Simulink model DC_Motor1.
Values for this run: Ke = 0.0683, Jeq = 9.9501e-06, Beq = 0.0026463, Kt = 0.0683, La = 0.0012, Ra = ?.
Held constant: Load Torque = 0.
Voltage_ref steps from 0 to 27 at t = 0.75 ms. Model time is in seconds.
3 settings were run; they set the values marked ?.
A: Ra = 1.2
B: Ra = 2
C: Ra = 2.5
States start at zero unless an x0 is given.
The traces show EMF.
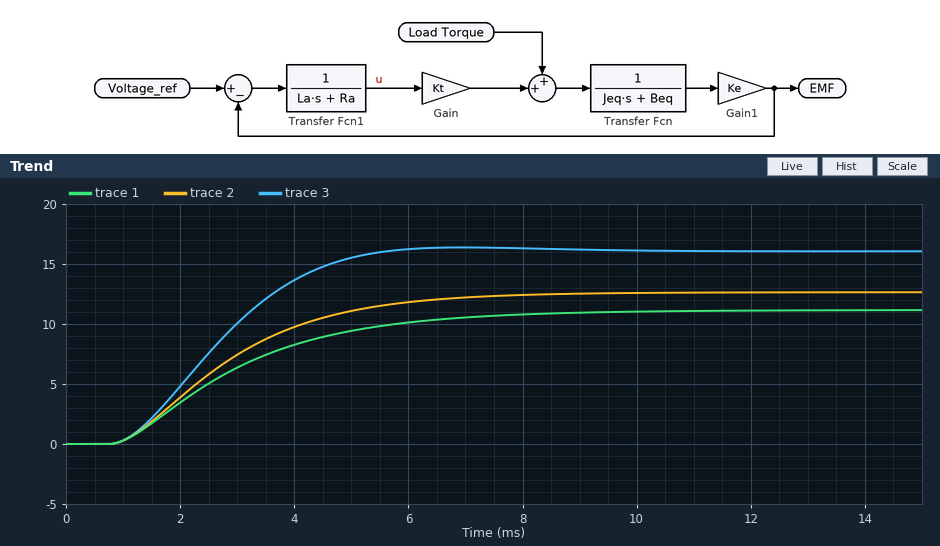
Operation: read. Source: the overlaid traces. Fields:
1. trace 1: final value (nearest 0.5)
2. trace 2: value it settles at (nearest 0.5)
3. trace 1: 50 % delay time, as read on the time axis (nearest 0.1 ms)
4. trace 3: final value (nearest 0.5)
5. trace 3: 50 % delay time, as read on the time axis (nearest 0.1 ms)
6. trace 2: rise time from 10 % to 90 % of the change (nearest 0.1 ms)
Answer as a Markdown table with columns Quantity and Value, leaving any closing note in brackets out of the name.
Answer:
| Quantity | Value |
|---|---|
| trace 1: final value | 11.0 |
| trace 2: value it settles at | 12.5 |
| trace 1: 50 % delay time, as read on the time axis | 2.7 ms |
| trace 3: final value | 16.0 |
| trace 3: 50 % delay time, as read on the time axis | 2.6 ms |
| trace 2: rise time from 10 % to 90 % of the change | 4.0 ms |
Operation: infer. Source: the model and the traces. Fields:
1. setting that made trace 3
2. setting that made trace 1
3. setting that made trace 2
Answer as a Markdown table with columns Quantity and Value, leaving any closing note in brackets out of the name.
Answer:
| Quantity | Value |
|---|---|
| setting that made trace 3 | A |
| setting that made trace 1 | C |
| setting that made trace 2 | B |
